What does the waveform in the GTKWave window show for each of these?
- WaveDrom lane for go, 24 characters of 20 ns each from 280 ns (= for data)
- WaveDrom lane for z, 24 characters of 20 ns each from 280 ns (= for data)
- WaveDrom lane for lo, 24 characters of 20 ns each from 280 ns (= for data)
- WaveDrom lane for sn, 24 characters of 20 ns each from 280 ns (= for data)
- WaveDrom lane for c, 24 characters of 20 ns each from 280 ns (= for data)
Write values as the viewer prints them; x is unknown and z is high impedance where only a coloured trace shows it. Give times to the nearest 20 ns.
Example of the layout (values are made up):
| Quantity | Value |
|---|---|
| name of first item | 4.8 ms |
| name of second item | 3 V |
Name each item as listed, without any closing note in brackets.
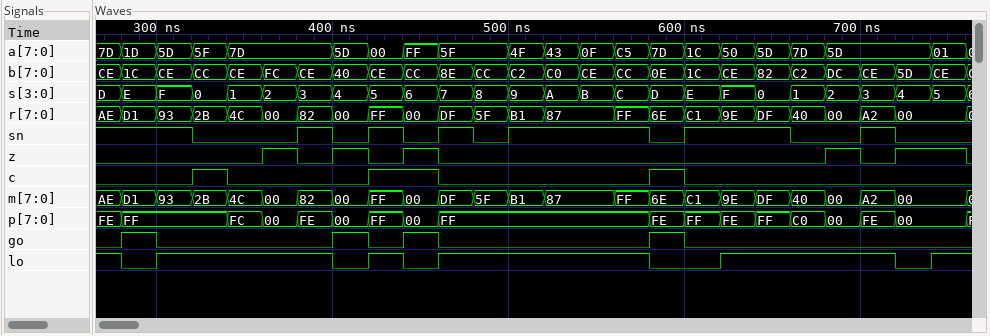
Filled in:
| Quantity | Value |
|---|---|
| WaveDrom lane for go, 24 characters of 20 ns each from 280 ns | {name: 'go', wave: '10....1010.....10.......'} |
| WaveDrom lane for z, 24 characters of 20 ns each from 280 ns | {name: 'z', wave: '0...101010..........101.'} |
| WaveDrom lane for lo, 24 characters of 20 ns each from 280 ns | {name: 'lo', wave: '01....0101.....0.1....01'} |
| WaveDrom lane for sn, 24 characters of 20 ns each from 280 ns | {name: 'sn', wave: '1.0..1010101...01..0.10.'} |
| WaveDrom lane for c, 24 characters of 20 ns each from 280 ns | {name: 'c', wave: '0.10...1.0.....10.......'} |
